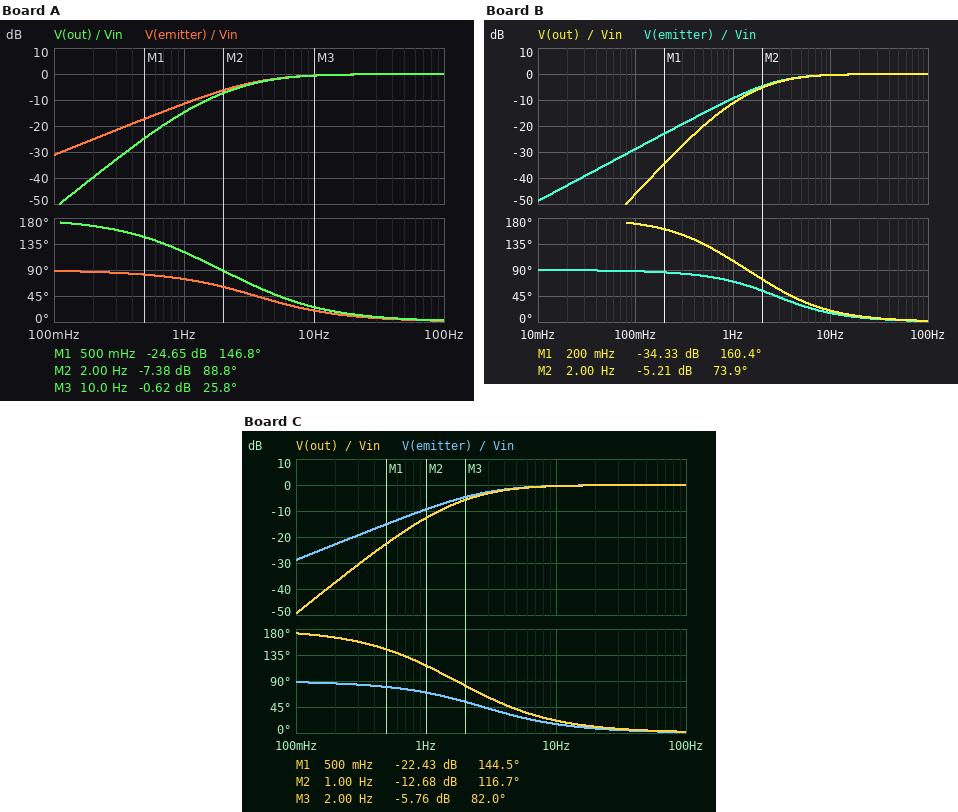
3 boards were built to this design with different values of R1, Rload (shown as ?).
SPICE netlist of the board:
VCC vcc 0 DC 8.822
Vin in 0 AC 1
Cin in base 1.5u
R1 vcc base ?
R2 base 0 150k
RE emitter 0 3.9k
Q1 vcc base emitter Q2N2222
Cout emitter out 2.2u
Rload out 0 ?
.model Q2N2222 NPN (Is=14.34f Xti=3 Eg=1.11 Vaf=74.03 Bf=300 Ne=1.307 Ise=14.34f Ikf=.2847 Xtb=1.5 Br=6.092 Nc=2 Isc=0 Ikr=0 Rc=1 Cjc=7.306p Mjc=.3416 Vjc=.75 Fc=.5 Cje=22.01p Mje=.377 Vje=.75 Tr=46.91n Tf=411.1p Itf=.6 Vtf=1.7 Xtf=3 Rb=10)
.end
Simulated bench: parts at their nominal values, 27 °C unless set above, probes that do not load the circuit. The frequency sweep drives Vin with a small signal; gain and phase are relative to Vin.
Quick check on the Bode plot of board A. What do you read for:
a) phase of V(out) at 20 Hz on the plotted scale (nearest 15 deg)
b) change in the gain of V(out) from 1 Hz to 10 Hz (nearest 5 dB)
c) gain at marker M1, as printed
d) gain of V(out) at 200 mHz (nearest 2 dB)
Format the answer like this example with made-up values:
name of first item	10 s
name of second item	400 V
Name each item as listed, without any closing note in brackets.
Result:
phase of V(out) at 20 Hz on the plotted scale	15 deg
change in the gain of V(out) from 1 Hz to 10 Hz	15 dB
gain at marker M1, as printed	-24.65 dB
gain of V(out) at 200 mHz	-40 dB
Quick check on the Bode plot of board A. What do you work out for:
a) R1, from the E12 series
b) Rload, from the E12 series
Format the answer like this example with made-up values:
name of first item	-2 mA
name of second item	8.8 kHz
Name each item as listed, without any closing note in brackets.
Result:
R1, from the E12 series	39 kΩ
Rload, from the E12 series	68 kΩ
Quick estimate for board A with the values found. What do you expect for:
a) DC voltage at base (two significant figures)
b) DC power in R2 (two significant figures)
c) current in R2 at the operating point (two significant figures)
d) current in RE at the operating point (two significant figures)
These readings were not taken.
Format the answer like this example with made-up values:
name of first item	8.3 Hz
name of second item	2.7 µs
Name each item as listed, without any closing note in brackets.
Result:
DC voltage at base	6.7 V
DC power in R2	300 µW
current in R2 at the operating point	45 µA
current in RE at the operating point	1.6 mA
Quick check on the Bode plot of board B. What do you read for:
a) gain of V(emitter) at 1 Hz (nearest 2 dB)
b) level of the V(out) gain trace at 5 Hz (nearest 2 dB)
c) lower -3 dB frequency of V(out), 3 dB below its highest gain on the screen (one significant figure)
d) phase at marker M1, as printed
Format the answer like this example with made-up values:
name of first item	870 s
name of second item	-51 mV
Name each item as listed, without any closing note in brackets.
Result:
gain of V(emitter) at 1 Hz	-10 dB
level of the V(out) gain trace at 5 Hz	-2 dB
lower -3 dB frequency of V(out), 3 dB below its highest gain on the screen	3 Hz
phase at marker M1, as printed	160.4 deg
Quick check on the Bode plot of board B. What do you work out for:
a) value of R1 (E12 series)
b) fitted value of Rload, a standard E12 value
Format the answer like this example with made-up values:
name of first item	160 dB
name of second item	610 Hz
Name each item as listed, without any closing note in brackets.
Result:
value of R1	56 kΩ
fitted value of Rload, a standard E12 value	100 kΩ
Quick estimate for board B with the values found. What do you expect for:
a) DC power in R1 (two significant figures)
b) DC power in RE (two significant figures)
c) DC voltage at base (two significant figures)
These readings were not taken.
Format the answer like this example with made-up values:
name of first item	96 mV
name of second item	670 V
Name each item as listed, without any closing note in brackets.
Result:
DC power in R1	130 µW
DC power in RE	7.6 mW
DC voltage at base	6.1 V
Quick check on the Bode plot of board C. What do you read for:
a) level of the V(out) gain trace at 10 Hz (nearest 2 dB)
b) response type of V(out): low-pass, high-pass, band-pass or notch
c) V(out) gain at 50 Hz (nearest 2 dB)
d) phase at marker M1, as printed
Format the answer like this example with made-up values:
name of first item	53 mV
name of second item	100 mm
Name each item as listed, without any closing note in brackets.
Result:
level of the V(out) gain trace at 10 Hz	0 dB
response type of V(out): low-pass, high-pass, band-pass or notch	high-pass
V(out) gain at 50 Hz	0 dB
phase at marker M1, as printed	144.5 deg
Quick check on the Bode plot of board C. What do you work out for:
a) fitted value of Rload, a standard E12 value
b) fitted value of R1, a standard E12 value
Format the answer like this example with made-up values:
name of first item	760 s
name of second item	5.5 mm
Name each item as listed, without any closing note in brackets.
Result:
fitted value of Rload, a standard E12 value	68 kΩ
fitted value of R1, a standard E12 value	56 kΩ
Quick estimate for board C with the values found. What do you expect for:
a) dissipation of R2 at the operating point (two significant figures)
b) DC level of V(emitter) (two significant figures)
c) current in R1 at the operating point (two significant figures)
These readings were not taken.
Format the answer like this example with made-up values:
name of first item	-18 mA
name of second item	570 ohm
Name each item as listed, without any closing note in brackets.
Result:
dissipation of R2 at the operating point	250 µW
DC level of V(emitter)	5.4 V
current in R1 at the operating point	49 µA
